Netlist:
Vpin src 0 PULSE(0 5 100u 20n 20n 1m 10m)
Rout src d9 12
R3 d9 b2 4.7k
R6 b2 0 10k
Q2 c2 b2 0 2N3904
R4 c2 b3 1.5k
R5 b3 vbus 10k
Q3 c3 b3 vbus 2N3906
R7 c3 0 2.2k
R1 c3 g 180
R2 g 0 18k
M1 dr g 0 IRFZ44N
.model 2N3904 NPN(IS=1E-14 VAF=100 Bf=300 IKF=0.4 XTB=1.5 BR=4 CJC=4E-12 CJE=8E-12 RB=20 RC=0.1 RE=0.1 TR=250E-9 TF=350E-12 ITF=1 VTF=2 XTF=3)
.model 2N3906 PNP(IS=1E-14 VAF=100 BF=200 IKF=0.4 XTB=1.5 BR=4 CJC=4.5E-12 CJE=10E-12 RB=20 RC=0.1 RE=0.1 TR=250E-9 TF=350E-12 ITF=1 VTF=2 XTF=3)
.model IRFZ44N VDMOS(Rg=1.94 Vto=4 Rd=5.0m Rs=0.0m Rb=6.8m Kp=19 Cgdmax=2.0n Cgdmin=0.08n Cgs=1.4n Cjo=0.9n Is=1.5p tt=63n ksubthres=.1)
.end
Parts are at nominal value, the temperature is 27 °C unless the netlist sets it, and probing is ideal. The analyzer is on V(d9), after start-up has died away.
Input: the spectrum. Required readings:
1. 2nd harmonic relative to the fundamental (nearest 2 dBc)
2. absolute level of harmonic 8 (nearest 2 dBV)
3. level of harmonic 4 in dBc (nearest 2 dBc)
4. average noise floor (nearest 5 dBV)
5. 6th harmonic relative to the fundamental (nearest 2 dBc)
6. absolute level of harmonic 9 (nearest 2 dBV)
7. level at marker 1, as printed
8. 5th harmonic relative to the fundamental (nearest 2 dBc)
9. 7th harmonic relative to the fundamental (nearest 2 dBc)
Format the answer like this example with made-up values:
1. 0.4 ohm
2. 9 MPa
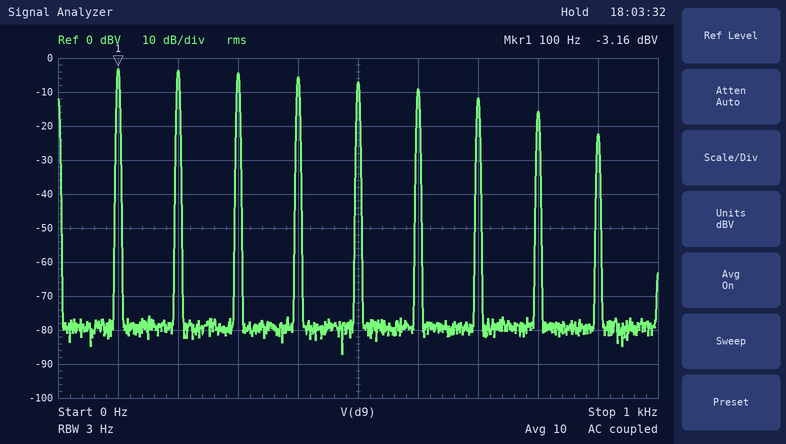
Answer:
1. 0 dBc
2. -16 dBV
3. -2 dBc
4. -80 dBV
5. -6 dBc
6. -22 dBV
7. -3.16 dBV
8. -4 dBc
9. -8 dBc
